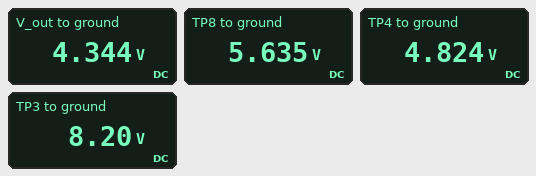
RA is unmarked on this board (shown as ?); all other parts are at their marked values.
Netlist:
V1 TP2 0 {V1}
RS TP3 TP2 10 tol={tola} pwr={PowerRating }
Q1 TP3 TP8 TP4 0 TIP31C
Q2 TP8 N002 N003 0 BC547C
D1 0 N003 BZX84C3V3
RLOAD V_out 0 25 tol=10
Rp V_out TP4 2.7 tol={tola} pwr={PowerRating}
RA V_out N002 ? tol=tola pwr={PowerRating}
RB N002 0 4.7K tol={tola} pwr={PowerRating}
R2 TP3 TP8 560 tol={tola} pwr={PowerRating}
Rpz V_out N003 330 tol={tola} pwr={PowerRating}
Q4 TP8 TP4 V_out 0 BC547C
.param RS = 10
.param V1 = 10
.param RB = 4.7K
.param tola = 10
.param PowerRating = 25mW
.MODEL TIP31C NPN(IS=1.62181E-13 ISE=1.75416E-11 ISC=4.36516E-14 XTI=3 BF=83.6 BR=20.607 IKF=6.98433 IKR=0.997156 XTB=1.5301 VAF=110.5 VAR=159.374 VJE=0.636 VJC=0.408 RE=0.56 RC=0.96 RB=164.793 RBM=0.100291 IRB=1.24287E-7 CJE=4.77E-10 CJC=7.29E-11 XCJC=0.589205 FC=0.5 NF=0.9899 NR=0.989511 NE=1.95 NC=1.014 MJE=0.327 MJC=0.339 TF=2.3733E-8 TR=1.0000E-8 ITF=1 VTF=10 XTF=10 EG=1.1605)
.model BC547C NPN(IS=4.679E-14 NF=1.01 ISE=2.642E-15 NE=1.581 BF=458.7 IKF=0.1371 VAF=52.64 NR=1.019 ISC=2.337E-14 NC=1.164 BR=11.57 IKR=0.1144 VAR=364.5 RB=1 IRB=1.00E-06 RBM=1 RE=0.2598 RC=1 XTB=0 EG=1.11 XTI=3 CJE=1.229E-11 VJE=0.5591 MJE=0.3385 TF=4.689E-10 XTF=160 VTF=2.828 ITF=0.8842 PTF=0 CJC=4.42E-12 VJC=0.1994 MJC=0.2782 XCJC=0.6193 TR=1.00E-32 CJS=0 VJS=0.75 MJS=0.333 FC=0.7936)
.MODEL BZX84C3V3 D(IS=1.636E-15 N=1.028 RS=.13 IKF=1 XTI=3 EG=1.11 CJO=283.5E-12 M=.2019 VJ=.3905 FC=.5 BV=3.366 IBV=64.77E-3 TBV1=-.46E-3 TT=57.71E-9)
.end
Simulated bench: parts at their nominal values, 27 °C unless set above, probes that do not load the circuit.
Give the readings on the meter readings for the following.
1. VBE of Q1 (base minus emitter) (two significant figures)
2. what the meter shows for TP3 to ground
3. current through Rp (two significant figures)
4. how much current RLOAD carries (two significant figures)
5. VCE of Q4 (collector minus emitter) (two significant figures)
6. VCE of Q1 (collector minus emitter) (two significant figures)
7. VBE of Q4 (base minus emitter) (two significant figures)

810 mV
8.20 V
180 mA
170 mA
1.3 V
3.4 V
480 mV
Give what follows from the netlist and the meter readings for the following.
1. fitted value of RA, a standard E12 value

470 Ω
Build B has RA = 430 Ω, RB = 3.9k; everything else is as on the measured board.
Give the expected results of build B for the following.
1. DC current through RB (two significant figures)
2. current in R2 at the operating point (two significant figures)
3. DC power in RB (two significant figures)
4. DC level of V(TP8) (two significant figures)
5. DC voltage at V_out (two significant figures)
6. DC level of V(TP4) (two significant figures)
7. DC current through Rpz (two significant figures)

1.0 mA
4.5 mA
4.0 mW
5.7 V
4.4 V
4.9 V
3.3 mA
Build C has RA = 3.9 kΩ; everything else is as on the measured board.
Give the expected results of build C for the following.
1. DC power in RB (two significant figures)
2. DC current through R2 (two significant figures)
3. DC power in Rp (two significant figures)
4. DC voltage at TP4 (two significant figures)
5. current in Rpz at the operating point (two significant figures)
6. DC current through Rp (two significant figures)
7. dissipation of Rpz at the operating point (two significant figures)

1.6 mW
2.6 mA
120 mW
5.6 V
5.3 mA
210 mA
9.3 mW
